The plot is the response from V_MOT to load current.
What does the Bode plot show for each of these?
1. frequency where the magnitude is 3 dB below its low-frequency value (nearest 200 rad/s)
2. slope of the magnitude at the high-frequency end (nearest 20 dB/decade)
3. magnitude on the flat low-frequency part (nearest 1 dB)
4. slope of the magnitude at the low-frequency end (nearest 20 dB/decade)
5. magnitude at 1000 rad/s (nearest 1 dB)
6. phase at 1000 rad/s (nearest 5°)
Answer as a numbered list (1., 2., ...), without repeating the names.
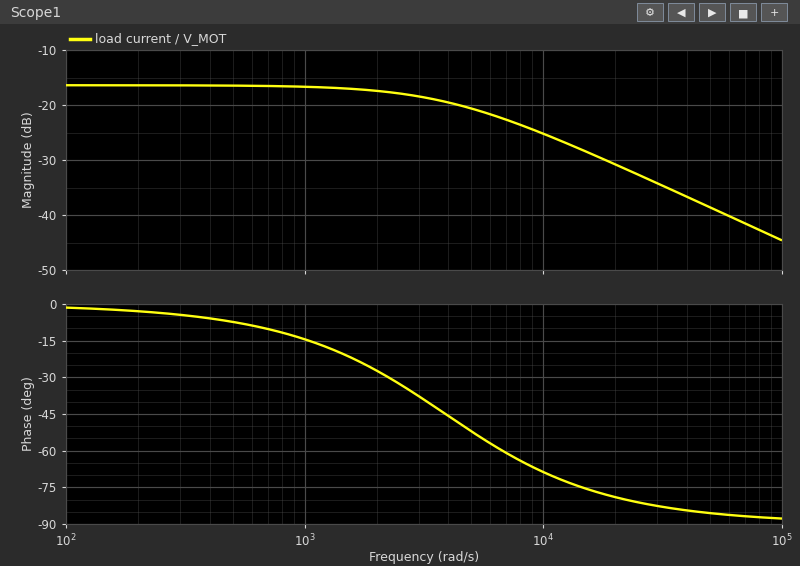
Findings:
1. 3800 rad/s
2. -20 dB/decade
3. -16 dB
4. 0 dB/decade
5. -17 dB
6. -15°
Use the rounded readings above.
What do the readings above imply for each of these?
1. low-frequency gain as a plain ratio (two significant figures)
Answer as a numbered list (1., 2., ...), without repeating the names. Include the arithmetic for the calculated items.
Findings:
1. 10^(-16 / 20) = 0.16
